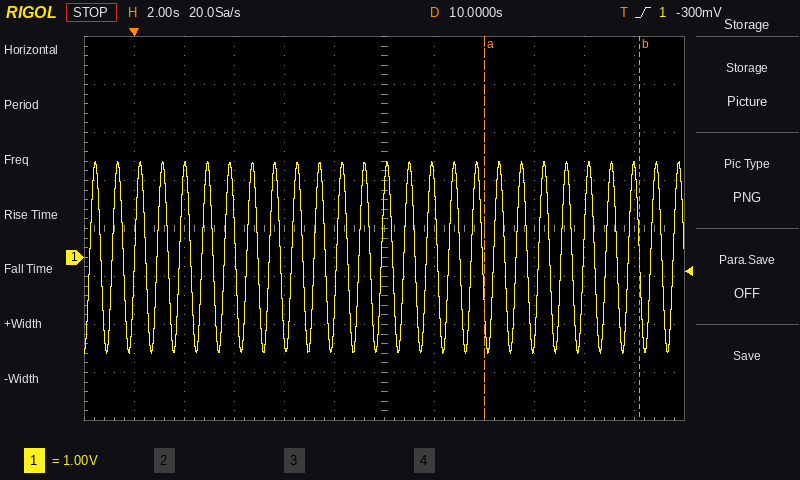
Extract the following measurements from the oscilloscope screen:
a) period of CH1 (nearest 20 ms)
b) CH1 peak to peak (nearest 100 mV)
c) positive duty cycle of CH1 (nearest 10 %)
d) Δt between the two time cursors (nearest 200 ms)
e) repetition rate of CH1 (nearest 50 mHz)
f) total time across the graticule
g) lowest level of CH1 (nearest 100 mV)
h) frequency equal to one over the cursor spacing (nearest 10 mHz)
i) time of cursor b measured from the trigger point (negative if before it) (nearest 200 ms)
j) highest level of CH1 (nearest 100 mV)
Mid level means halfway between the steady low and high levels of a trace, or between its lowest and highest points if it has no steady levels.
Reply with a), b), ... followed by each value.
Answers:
a) 900 ms
b) 4.0 V
c) 50 %
d) 6.2 s
e) 1.10 Hz
f) 24 s
g) -2.0 V
h) 160 mHz
i) +20.2 s
j) 2.0 V
